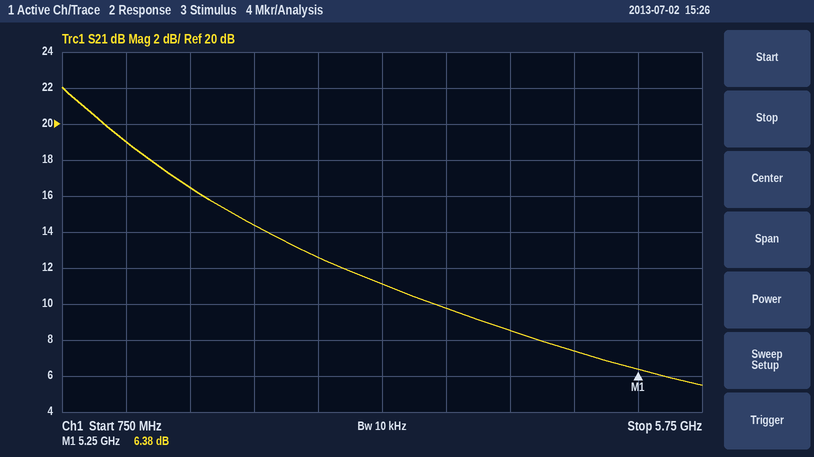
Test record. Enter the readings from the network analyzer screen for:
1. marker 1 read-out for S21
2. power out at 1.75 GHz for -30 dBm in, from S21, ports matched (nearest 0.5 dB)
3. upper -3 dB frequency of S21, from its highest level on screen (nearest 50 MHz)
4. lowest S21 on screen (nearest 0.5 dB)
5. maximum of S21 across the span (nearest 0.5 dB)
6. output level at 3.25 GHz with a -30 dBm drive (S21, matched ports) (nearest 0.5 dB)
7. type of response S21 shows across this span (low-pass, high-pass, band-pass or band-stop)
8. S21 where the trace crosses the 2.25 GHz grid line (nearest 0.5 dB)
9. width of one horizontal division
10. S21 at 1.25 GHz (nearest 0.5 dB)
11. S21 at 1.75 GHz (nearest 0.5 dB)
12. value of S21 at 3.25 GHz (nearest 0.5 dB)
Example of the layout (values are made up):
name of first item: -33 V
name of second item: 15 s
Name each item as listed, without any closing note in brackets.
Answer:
marker 1 read-out for S21: 6.38 dB
power out at 1.75 GHz for -30 dBm in, from S21, ports matched: -13.5 dBm
upper -3 dB frequency of S21, from its highest level on screen: 1.25 GHz
lowest S21 on screen: 5.5 dB
maximum of S21 across the span: 22.0 dB
output level at 3.25 GHz with a -30 dBm drive (S21, matched ports): -19.0 dBm
type of response S21 shows across this span: low-pass
S21 where the trace crosses the 2.25 GHz grid line: 14.5 dB
width of one horizontal division: 500 MHz
S21 at 1.25 GHz: 19.0 dB
S21 at 1.75 GHz: 16.5 dB
value of S21 at 3.25 GHz: 11.0 dB
